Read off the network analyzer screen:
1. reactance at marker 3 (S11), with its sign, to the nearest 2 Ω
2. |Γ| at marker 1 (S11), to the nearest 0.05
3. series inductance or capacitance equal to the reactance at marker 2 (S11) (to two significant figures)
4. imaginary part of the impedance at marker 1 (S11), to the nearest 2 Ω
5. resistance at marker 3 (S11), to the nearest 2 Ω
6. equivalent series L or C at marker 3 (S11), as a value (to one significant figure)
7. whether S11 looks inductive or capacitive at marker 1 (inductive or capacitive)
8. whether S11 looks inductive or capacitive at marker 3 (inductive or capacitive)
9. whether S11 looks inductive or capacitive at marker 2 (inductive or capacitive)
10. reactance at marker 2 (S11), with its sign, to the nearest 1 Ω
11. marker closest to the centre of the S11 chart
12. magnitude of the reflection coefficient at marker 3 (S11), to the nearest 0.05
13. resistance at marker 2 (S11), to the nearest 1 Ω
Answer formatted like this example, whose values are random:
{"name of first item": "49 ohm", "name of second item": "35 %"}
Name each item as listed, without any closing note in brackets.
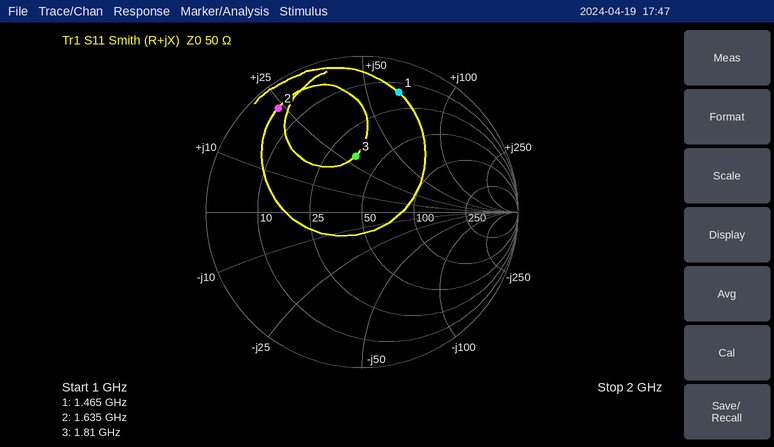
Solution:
{"reactance at marker 3 (S11), with its sign, to the nearest 2 Ω": "+30 Ω", "|Γ| at marker 1 (S11), to the nearest 0.05": "0.80", "series inductance or capacitance equal to the reactance at marker 2 (S11)": "2.3 nH", "imaginary part of the impedance at marker 1 (S11), to the nearest 2 Ω": "+66 Ω", "resistance at marker 3 (S11), to the nearest 2 Ω": "36 Ω", "equivalent series L or C at marker 3 (S11), as a value": "3 nH", "whether S11 looks inductive or capacitive at marker 1": "inductive", "whether S11 looks inductive or capacitive at marker 3": "inductive", "whether S11 looks inductive or capacitive at marker 2": "inductive", "reactance at marker 2 (S11), with its sign, to the nearest 1 Ω": "+24 Ω", "marker closest to the centre of the S11 chart": "marker 3", "magnitude of the reflection coefficient at marker 3 (S11), to the nearest 0.05": "0.35", "resistance at marker 2 (S11), to the nearest 1 Ω": "5 Ω"}
